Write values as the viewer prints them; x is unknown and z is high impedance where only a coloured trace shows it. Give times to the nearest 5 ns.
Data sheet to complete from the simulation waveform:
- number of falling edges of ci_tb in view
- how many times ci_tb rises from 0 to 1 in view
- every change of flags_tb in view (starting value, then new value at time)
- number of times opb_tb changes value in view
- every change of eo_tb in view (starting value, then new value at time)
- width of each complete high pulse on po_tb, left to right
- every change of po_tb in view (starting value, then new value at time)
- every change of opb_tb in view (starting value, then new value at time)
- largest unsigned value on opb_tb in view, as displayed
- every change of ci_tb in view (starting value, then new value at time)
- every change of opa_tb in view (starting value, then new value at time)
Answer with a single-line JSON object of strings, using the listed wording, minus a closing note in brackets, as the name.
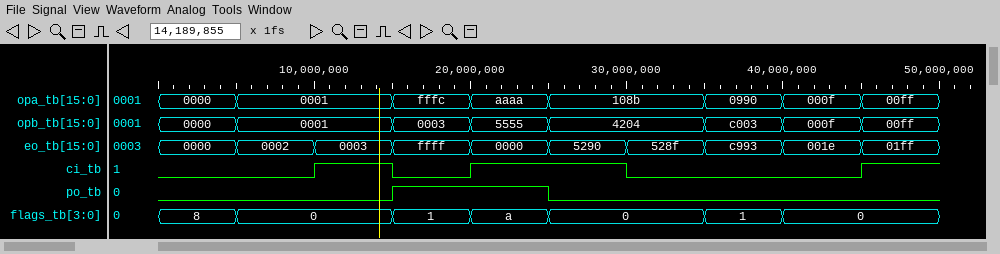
{"number of falling edges of ci_tb in view": "2", "how many times ci_tb rises from 0 to 1 in view": "3", "every change of flags_tb in view": "8, 0 at 5 ns, 1 at 15 ns, a at 20 ns, 0 at 25 ns, 1 at 35 ns, 0 at 40 ns", "number of times opb_tb changes value in view": "7", "every change of eo_tb in view": "0000, 0002 at 5 ns, 0003 at 10 ns, ffff at 15 ns, 0000 at 20 ns, 5290 at 25 ns, 528f at 30 ns, c993 at 35 ns, 001e at 40 ns, 01ff at 45 ns", "width of each complete high pulse on po_tb, left to right": "10 ns", "every change of po_tb in view": "0, 1 at 15 ns, 0 at 25 ns", "every change of opb_tb in view": "0000, 0001 at 5 ns, 0003 at 15 ns, 5555 at 20 ns, 4204 at 25 ns, c003 at 35 ns, 000f at 40 ns, 00ff at 45 ns", "largest unsigned value on opb_tb in view, as displayed": "c003", "every change of ci_tb in view": "0, 1 at 10 ns, 0 at 15 ns, 1 at 20 ns, 0 at 30 ns, 1 at 45 ns", "every change of opa_tb in view": "0000, 0001 at 5 ns, fffc at 15 ns, aaaa at 20 ns, 108b at 25 ns, 0990 at 35 ns, 000f at 40 ns, 00ff at 45 ns"}
